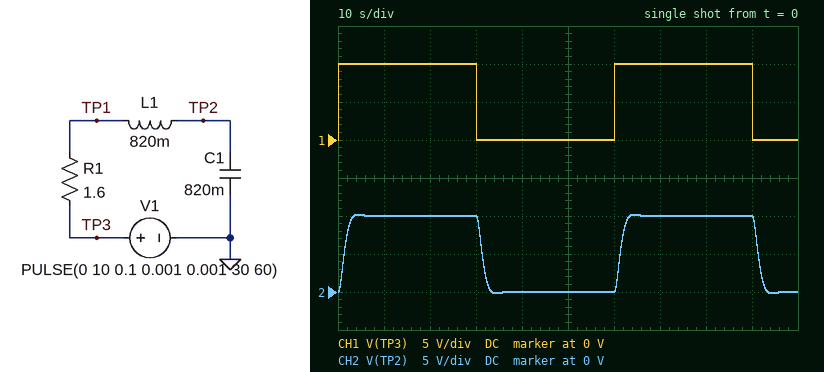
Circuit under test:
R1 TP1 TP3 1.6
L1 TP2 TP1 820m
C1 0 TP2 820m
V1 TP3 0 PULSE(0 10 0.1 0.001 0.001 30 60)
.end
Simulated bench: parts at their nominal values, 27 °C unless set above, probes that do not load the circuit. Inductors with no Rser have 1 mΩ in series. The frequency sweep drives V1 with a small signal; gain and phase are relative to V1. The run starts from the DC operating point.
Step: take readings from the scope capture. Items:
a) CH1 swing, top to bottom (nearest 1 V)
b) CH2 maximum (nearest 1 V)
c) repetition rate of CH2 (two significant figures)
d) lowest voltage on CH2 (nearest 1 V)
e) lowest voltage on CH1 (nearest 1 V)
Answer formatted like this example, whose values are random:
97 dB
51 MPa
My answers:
10 V
10 V
17 mHz
0 V
0 V
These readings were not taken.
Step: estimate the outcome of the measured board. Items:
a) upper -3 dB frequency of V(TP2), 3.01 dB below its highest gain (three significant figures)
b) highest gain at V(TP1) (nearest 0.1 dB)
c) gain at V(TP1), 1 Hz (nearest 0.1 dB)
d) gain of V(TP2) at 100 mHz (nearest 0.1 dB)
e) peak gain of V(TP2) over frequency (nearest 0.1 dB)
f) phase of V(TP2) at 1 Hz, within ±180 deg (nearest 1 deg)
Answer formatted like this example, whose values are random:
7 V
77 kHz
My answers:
169 mHz
0 dB
-0.4 dB
-0.9 dB
0 dB
-162 deg
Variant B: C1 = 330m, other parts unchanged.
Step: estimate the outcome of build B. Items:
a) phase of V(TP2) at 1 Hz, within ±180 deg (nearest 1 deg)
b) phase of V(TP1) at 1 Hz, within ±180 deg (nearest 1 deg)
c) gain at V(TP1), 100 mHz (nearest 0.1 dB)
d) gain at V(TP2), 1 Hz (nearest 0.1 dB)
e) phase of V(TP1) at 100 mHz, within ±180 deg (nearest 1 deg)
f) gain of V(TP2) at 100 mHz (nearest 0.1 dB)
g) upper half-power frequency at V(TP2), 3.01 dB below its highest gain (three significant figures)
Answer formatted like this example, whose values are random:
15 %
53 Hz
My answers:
-161 deg
19 deg
-0.6 dB
-20.2 dB
-20 deg
0.4 dB
357 mHz
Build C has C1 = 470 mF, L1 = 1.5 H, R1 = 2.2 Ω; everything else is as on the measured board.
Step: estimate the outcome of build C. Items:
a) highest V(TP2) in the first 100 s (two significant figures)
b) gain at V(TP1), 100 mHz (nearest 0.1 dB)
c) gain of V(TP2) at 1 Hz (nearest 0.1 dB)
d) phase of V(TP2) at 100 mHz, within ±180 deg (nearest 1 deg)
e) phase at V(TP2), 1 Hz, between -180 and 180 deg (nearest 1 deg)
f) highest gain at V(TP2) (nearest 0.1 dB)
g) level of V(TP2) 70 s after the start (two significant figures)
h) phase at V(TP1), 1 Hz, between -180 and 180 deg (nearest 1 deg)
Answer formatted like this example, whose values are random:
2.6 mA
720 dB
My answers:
11 V
-2.6 dB
-28.8 dB
-42 deg
-166 deg
0.3 dB
10 V
14 deg
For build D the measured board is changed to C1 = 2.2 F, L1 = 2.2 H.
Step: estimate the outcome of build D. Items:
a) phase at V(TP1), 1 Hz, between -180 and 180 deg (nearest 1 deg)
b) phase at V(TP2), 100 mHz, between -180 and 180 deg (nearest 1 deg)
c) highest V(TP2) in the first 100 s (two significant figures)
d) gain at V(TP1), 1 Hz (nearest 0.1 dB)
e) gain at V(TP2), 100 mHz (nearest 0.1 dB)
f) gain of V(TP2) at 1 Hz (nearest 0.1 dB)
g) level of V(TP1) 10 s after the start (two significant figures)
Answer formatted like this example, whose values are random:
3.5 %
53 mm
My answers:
7 deg
-112 deg
10 V
-0.1 dB
-7.6 dB
-45.6 dB
9.7 V
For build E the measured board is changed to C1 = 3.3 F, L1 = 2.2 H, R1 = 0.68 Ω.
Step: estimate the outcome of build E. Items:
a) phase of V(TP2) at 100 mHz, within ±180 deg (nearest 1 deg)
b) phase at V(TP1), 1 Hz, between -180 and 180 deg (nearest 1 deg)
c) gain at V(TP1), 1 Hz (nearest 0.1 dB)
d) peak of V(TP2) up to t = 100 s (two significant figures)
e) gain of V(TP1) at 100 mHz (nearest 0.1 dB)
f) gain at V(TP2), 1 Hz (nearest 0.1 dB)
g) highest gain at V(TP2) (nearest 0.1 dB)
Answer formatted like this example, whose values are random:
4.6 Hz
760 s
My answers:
-143 deg
3 deg
0 dB
12 V
-2.0 dB
-49.1 dB
2.4 dB
